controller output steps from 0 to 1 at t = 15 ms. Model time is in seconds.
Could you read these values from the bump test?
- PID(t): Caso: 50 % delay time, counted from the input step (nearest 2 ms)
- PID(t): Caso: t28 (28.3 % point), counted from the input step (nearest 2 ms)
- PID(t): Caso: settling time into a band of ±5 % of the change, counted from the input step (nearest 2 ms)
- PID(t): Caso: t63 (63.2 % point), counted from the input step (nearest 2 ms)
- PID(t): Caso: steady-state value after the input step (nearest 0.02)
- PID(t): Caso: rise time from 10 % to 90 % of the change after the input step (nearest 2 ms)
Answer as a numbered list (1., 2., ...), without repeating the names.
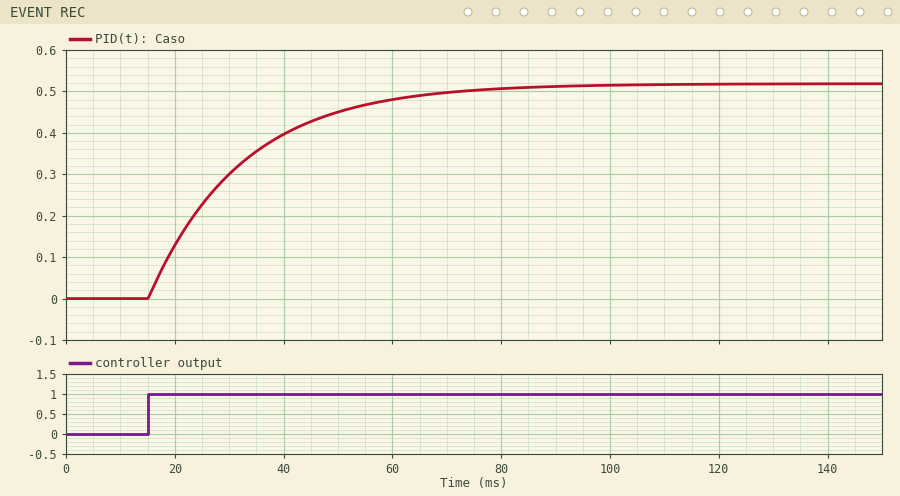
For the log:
1. 12 ms
2. 6 ms
3. 52 ms
4. 18 ms
5. 0.52
6. 38 ms
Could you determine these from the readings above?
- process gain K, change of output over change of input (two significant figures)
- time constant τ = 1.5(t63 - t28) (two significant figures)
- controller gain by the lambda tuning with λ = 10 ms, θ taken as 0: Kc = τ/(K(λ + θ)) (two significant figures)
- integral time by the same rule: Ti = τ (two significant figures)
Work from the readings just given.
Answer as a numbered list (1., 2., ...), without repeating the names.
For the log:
1. 0.52
2. 18 ms
3. 3.5
4. 18 ms
